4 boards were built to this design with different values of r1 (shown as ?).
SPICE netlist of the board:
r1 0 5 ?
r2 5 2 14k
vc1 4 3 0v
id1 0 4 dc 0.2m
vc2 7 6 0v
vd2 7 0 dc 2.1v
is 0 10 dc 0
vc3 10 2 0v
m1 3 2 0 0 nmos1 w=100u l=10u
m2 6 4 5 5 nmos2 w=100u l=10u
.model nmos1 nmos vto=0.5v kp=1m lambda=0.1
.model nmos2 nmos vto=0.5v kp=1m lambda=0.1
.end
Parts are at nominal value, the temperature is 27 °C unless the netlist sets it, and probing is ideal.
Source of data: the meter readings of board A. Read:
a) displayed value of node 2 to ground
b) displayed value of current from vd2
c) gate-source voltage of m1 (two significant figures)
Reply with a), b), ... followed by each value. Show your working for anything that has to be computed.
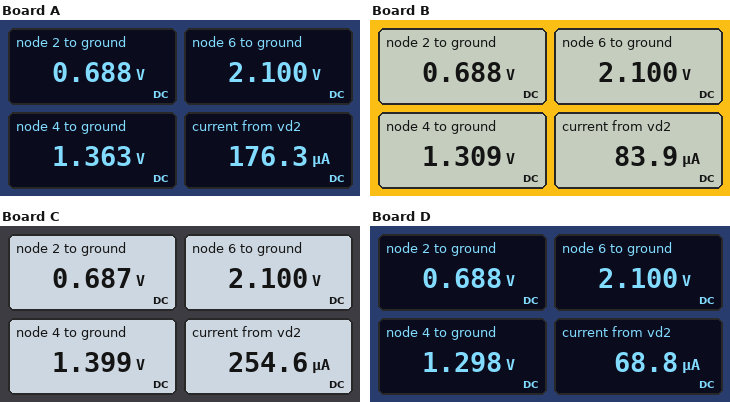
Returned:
a) 0.688 V
b) 176.3 µA
c) 688 mV = 690 mV
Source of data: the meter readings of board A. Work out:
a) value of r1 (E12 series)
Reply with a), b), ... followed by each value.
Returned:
a) 3.9 kΩ
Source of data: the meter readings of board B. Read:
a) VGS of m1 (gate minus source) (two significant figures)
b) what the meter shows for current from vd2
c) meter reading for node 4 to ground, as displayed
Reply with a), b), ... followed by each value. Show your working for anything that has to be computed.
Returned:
a) 688 mV = 690 mV
b) 83.9 µA
c) 1.309 V
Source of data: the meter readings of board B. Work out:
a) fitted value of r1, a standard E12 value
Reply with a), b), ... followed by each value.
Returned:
a) 8.2 kΩ
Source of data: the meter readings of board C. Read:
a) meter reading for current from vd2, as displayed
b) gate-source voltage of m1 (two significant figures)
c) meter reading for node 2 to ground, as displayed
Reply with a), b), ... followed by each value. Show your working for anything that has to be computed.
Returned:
a) 254.6 µA
b) 687 mV = 690 mV
c) 0.687 V
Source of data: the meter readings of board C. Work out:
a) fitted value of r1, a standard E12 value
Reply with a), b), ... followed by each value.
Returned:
a) 2.7 kΩ
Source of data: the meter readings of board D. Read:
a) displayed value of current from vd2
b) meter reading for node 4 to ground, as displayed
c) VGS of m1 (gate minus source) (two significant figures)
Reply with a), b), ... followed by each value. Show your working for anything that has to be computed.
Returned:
a) 68.8 µA
b) 1.298 V
c) 688 mV = 690 mV
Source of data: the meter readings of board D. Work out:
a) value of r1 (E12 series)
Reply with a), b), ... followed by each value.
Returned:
a) 10 kΩ
